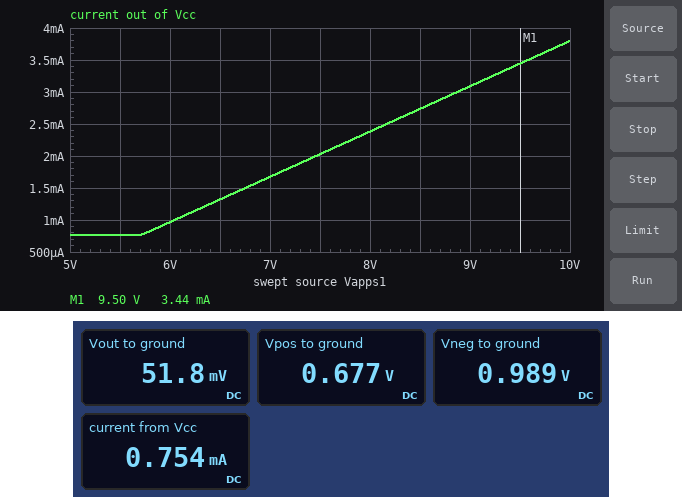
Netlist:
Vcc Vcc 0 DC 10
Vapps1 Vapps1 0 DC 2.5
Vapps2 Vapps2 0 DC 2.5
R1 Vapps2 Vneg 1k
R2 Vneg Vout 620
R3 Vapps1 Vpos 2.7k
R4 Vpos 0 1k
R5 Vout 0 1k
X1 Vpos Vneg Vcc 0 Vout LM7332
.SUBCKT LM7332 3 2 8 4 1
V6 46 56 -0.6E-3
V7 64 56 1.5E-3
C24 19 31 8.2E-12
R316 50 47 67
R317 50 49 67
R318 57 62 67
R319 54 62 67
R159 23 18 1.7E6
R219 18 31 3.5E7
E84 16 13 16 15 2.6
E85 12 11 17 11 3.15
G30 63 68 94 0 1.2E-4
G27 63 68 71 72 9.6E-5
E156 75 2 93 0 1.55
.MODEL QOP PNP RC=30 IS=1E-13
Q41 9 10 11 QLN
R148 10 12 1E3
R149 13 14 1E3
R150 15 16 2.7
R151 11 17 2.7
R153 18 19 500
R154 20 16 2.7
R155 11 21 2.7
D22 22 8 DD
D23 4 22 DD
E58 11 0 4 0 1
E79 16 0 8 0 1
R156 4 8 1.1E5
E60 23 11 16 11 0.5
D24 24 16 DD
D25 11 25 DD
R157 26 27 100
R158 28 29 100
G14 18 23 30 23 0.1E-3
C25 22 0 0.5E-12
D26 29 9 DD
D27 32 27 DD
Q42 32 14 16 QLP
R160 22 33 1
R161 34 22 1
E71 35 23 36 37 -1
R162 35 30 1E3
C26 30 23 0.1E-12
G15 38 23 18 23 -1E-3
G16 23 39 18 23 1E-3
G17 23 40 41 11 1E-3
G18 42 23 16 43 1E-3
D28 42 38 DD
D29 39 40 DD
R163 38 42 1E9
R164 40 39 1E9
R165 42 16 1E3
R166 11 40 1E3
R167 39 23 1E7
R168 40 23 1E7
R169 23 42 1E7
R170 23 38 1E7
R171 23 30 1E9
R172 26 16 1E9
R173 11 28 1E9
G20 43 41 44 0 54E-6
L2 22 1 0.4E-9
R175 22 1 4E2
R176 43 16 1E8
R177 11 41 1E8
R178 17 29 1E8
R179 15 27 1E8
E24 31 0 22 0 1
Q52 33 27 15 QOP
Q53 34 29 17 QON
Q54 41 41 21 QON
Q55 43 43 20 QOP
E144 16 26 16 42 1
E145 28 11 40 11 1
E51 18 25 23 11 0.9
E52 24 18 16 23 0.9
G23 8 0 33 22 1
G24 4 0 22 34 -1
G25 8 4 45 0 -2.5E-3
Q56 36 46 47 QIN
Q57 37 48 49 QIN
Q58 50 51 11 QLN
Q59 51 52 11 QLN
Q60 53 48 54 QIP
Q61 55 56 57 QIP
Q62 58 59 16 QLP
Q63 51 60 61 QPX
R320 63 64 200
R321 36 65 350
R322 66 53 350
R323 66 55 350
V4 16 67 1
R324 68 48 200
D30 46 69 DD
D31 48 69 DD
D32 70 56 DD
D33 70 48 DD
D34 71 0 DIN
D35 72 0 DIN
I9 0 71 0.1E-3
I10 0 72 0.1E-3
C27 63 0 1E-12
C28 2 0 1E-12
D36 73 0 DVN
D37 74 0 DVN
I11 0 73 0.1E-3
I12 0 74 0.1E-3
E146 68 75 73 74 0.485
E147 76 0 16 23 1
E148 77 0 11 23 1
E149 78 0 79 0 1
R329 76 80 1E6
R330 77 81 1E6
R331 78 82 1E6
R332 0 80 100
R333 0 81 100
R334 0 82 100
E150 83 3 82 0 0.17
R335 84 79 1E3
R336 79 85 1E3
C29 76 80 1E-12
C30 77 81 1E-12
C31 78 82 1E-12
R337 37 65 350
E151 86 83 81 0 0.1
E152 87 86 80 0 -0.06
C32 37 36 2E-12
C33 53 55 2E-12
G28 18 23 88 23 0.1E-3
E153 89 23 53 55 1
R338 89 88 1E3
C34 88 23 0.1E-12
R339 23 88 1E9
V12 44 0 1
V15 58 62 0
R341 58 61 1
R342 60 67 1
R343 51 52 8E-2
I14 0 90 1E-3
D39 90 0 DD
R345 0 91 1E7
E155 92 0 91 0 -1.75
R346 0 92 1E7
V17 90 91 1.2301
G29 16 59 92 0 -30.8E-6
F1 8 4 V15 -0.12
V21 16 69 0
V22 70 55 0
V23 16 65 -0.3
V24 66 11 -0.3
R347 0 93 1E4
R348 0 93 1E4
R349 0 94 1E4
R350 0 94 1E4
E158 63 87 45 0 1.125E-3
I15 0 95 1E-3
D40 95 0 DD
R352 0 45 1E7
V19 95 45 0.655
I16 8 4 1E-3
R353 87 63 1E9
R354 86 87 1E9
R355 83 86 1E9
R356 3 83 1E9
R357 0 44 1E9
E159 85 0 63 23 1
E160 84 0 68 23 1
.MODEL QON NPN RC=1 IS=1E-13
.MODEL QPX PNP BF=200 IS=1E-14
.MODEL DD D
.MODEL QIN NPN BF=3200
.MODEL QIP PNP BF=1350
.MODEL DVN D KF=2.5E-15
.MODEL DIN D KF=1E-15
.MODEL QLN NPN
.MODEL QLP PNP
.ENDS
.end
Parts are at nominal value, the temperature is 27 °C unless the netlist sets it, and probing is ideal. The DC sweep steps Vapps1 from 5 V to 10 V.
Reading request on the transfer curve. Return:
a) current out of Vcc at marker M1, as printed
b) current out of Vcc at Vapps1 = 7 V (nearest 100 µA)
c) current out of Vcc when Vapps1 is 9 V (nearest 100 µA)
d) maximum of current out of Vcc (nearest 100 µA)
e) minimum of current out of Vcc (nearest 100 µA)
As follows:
3.44 mA
1.7 mA
3.1 mA
3.8 mA
800 µA
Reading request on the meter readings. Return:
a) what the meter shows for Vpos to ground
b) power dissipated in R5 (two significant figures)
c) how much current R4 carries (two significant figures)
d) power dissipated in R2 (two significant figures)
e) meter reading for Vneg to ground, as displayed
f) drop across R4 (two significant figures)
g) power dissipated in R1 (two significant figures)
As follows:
0.677 V
2.7 µW
680 µA
1.4 mW
0.989 V
680 mV
2.3 mW
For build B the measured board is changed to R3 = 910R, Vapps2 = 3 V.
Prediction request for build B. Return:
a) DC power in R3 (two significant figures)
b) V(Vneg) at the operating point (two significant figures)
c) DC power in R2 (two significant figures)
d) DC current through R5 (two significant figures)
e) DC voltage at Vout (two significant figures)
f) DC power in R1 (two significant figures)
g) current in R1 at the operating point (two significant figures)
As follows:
1.6 mW
1.3 V
1.8 mW
260 µA
260 mV
2.9 mW
1.7 mA
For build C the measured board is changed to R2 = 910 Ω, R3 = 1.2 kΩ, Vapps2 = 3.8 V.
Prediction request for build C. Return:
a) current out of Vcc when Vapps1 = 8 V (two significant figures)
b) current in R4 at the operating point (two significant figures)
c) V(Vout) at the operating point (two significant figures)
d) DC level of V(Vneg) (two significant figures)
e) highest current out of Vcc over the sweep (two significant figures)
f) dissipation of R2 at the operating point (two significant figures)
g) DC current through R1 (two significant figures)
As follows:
4.1 mA
1.1 mA
54 mV
1.8 V
6.7 mA
3.5 mW
2.0 mA
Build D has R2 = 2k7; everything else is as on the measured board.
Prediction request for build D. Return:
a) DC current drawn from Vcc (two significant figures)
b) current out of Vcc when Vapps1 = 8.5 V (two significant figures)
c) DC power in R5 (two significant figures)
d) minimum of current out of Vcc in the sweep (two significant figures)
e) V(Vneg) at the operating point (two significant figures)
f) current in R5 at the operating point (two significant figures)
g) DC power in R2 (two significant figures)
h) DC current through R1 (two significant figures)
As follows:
750 µA
2.3 mA
2.2 µW
750 µA
1.8 V
47 µA
1.2 mW
660 µA
